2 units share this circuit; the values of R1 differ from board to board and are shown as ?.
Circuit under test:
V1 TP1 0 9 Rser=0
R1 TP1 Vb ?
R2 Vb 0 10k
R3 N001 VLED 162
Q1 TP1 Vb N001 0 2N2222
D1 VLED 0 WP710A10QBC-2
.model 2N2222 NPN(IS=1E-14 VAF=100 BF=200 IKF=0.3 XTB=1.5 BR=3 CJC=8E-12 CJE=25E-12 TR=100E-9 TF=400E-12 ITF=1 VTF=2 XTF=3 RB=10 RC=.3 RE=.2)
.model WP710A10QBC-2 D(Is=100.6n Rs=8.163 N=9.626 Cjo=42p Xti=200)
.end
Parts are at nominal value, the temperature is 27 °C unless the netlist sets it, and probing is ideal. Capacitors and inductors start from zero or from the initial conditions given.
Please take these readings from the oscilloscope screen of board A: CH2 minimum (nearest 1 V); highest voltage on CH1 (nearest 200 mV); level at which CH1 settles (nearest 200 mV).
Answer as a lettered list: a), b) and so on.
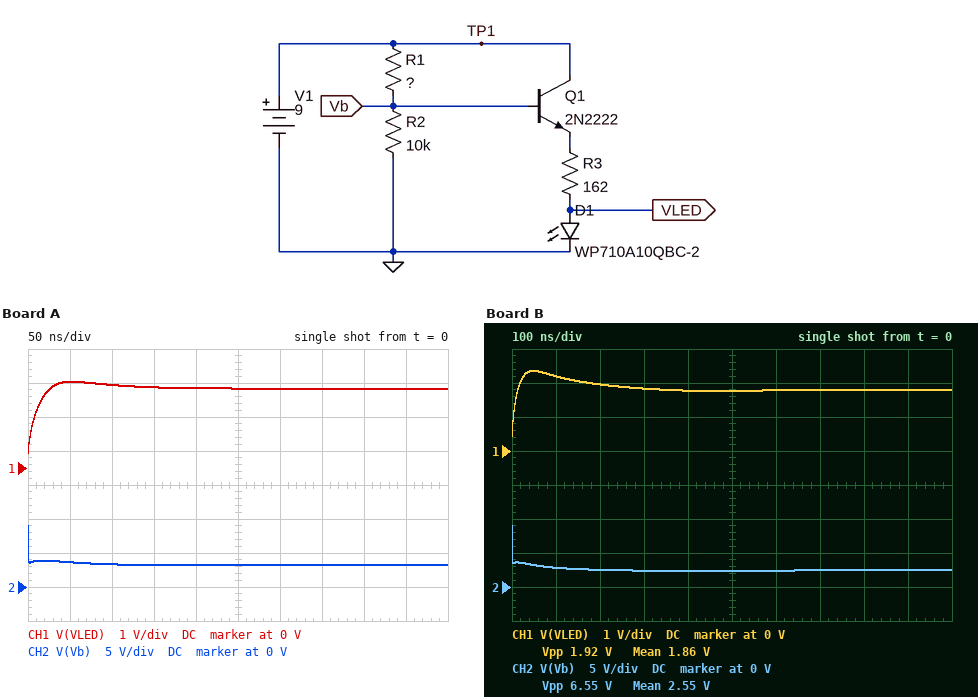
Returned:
a) 3 V
b) 2.6 V
c) 2.4 V
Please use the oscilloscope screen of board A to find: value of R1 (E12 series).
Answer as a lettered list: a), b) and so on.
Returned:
a) 18 kΩ
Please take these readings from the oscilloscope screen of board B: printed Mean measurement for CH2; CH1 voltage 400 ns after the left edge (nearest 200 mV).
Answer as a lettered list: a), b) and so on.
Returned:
a) 2.55 V
b) 1.8 V
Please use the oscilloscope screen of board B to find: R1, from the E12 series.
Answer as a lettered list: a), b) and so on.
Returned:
a) 27 kΩ
